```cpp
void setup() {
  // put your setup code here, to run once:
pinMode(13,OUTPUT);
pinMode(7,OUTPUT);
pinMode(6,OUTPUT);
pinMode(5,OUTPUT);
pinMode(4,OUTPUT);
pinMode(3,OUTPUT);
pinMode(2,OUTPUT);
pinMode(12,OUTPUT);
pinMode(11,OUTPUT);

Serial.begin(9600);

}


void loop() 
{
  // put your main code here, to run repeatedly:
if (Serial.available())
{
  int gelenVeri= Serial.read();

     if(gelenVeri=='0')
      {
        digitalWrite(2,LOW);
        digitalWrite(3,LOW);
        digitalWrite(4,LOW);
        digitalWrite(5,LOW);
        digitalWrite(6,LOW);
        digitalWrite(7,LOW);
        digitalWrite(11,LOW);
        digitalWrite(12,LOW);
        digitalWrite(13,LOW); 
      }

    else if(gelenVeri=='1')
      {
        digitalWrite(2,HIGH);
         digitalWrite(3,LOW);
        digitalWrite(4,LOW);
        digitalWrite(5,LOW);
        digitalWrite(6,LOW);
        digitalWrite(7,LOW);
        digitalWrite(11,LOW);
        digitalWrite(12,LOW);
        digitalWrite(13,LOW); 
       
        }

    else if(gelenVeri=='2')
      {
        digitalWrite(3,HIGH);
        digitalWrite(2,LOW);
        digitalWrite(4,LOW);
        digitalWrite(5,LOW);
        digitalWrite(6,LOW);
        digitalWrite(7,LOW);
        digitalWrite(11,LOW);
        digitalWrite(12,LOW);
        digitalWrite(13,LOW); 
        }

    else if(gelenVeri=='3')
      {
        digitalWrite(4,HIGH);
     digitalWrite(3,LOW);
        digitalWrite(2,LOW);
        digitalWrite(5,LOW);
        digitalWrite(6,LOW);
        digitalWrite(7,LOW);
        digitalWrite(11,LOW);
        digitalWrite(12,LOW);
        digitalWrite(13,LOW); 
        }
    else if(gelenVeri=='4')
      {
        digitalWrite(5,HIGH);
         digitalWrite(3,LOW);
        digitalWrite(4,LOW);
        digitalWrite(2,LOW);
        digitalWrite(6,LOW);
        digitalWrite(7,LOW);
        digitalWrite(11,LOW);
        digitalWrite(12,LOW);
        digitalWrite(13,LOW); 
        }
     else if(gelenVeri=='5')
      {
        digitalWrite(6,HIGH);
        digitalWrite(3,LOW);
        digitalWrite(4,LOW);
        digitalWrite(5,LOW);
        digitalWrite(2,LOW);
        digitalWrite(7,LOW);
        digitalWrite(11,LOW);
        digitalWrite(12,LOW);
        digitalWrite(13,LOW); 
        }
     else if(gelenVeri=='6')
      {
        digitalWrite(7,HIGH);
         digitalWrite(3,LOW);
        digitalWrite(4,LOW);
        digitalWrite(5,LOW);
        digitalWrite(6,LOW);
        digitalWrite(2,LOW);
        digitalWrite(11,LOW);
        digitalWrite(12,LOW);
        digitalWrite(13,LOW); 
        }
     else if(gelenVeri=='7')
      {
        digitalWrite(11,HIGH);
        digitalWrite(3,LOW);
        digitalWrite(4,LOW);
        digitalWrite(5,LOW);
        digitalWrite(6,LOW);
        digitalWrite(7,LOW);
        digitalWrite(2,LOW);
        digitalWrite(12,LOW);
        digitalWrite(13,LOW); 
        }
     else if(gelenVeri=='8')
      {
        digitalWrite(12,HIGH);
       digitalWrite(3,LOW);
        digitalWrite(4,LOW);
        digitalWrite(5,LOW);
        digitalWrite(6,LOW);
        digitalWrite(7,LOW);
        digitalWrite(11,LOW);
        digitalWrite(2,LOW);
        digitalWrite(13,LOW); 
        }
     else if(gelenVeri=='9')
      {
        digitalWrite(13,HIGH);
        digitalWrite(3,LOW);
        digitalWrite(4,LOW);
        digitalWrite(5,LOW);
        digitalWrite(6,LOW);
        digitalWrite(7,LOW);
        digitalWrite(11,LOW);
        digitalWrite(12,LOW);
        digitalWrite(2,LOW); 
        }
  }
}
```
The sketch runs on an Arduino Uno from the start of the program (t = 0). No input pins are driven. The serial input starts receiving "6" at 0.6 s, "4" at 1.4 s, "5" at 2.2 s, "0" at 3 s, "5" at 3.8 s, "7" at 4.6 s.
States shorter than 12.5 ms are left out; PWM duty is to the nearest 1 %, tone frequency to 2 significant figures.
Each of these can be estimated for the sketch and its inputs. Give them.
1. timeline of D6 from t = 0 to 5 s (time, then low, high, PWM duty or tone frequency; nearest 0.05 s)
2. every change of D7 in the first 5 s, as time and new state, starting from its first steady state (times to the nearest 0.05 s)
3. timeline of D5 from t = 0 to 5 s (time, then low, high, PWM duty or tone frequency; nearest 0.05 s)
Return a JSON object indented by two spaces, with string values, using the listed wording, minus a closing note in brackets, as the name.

{
  "timeline of D6 from t = 0 to 5 s": "0 s low; 2.2 s high; 3 s low; 3.8 s high; 4.6 s low",
  "every change of D7 in the first 5 s, as time and new state, starting from its first steady state": "0 s low; 0.6 s high; 1.4 s low",
  "timeline of D5 from t = 0 to 5 s": "0 s low; 1.4 s high; 2.2 s low"
}
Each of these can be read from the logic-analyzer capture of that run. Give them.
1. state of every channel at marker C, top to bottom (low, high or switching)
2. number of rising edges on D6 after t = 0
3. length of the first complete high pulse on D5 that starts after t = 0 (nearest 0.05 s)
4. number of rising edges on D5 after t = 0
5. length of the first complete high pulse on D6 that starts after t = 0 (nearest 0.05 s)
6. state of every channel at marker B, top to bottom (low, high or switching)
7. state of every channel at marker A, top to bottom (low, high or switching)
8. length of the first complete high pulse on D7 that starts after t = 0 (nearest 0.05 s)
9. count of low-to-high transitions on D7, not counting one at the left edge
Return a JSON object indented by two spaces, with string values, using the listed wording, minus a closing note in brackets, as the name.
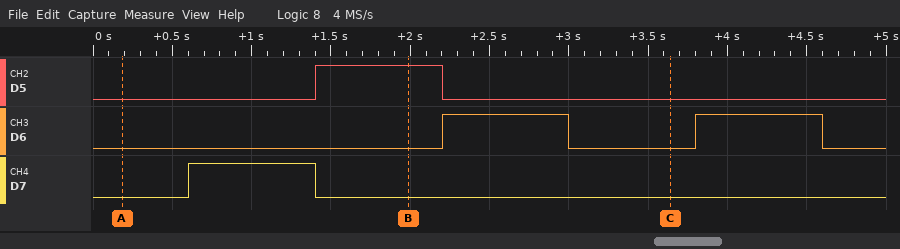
{
  "state of every channel at marker C, top to bottom": "D5 low, D6 low, D7 low",
  "number of rising edges on D6 after t = 0": "2",
  "length of the first complete high pulse on D5 that starts after t = 0": "0.80 s",
  "number of rising edges on D5 after t = 0": "1",
  "length of the first complete high pulse on D6 that starts after t = 0": "0.80 s",
  "state of every channel at marker B, top to bottom": "D5 high, D6 low, D7 low",
  "state of every channel at marker A, top to bottom": "D5 low, D6 low, D7 low",
  "length of the first complete high pulse on D7 that starts after t = 0": "0.80 s",
  "count of low-to-high transitions on D7, not counting one at the left edge": "1"
}
